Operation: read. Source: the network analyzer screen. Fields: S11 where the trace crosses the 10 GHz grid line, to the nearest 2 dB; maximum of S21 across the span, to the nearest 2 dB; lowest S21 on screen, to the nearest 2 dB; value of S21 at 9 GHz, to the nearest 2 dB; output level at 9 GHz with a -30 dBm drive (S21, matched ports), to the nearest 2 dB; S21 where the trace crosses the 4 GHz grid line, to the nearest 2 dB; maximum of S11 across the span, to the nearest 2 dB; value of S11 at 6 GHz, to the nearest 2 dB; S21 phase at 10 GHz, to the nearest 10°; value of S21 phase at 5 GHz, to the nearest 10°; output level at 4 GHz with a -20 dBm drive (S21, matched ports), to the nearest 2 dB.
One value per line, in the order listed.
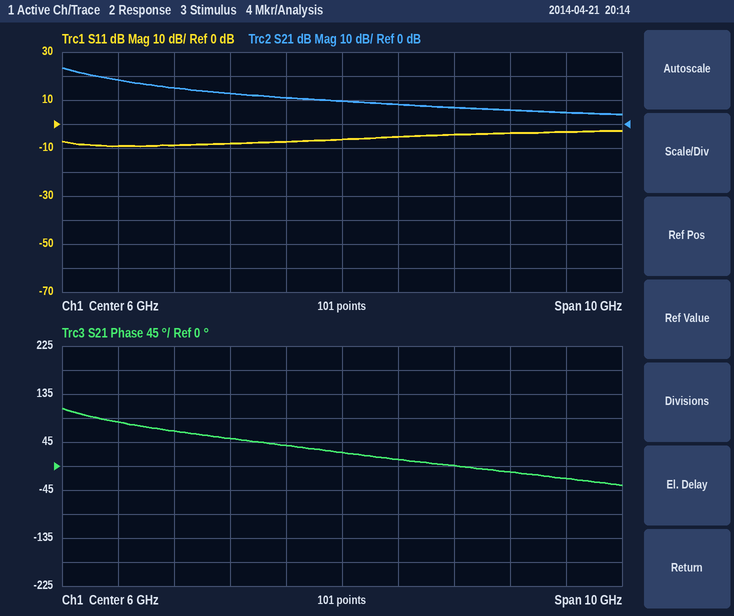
-4 dB
24 dB
4 dB
6 dB
-24 dBm
12 dB
-2 dB
-6 dB
-20°
40°
-8 dBm
